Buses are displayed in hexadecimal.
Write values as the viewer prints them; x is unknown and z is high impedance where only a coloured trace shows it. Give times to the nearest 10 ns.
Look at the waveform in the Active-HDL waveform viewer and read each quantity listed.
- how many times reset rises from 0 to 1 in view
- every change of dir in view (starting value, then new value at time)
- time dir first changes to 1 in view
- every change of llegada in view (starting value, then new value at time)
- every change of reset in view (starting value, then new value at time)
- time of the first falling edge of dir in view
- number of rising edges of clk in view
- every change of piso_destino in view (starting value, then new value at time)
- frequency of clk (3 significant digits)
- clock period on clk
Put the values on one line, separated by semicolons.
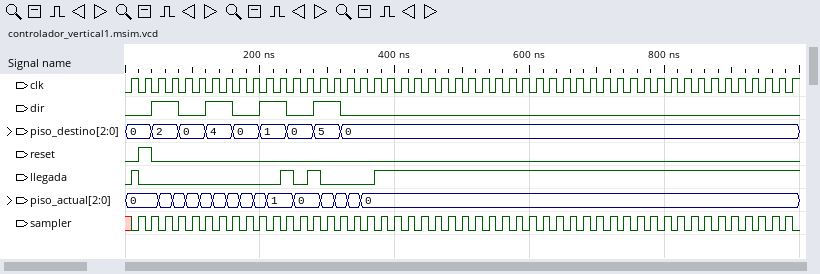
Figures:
1; 0, 1 at 40 ns, 0 at 80 ns, 1 at 120 ns, 0 at 160 ns, 1 at 200 ns, 0 at 240 ns, 1 at 280 ns, 0 at 320 ns; 40 ns; 0, 1 at 10 ns, 0 at 20 ns, 1 at 230 ns, 0 at 250 ns, 1 at 270 ns, 0 at 290 ns, 1 at 370 ns; 0, 1 at 20 ns, 0 at 40 ns; 80 ns; 50; 0, 2 at 40 ns, 0 at 80 ns, 4 at 120 ns, 0 at 160 ns, 1 at 200 ns, 0 at 240 ns, 5 at 280 ns, 0 at 320 ns; 50.0 MHz; 20 ns
